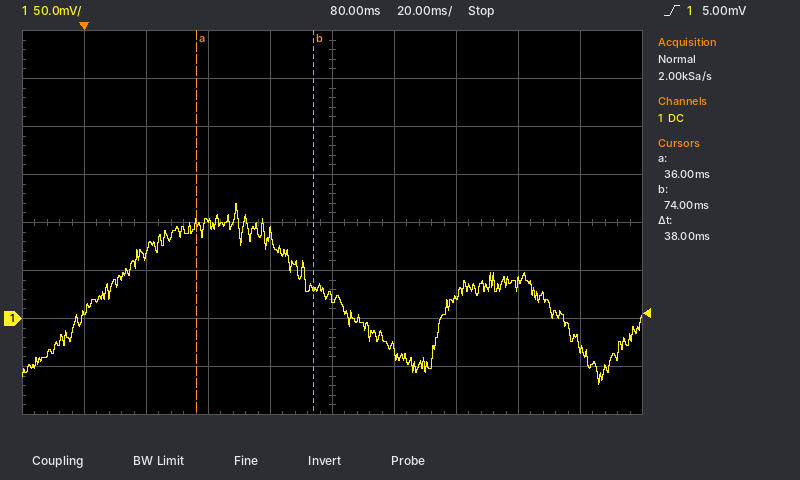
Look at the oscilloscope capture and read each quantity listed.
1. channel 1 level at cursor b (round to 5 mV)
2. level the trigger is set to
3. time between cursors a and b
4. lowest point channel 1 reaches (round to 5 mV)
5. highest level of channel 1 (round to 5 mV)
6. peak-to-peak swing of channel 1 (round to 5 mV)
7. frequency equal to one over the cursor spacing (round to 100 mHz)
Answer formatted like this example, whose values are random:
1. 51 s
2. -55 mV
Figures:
1. 30 mV
2. 5.00 mV
3. 38 ms
4. -70 mV
5. 120 mV
6. 190 mV
7. 26.3 Hz
